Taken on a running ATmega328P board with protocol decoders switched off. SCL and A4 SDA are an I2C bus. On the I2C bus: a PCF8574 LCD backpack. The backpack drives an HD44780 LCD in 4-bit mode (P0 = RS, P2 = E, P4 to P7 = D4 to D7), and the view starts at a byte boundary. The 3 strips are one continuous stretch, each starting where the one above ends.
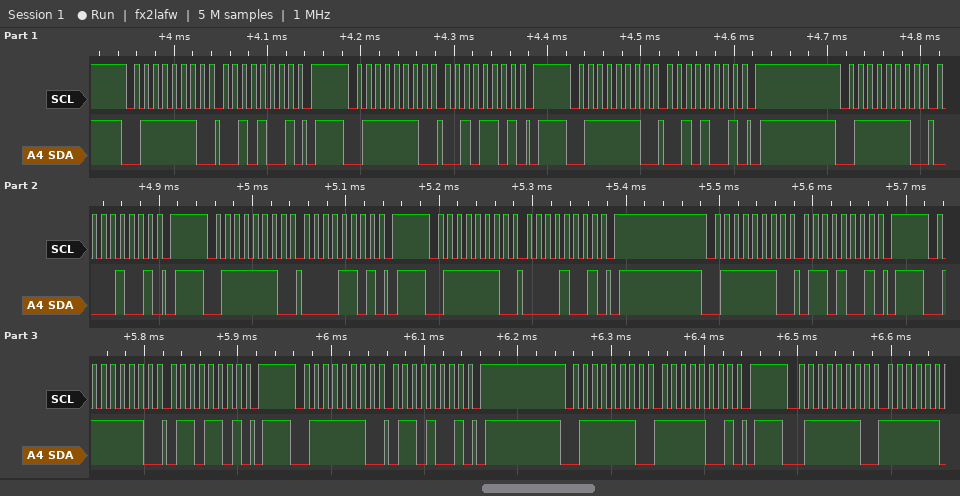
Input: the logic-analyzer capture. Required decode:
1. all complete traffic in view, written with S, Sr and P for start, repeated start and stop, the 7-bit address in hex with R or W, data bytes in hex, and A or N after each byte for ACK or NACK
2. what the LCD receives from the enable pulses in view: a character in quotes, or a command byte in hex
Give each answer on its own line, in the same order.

S 3FW A 29 A P S 3FW A 2D A P S 3FW A 29 A P S 3FW A 09 A P S 3FW A 0D A P S 3FW A 09 A P S 3FW A 69 A P S 3FW A 6D A P S 3FW A 69 A P S 3FW A F9 A P S 3FW A
' '
